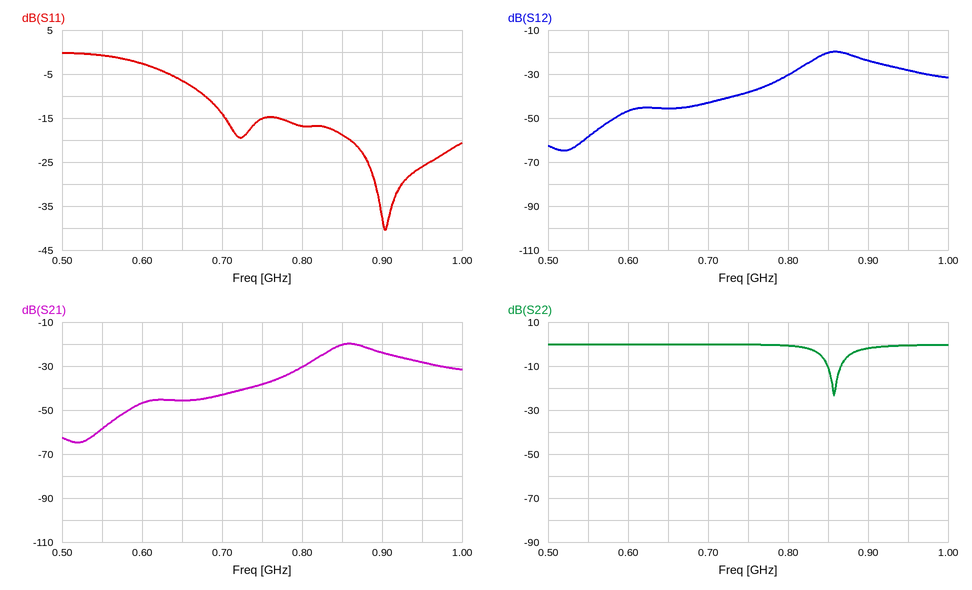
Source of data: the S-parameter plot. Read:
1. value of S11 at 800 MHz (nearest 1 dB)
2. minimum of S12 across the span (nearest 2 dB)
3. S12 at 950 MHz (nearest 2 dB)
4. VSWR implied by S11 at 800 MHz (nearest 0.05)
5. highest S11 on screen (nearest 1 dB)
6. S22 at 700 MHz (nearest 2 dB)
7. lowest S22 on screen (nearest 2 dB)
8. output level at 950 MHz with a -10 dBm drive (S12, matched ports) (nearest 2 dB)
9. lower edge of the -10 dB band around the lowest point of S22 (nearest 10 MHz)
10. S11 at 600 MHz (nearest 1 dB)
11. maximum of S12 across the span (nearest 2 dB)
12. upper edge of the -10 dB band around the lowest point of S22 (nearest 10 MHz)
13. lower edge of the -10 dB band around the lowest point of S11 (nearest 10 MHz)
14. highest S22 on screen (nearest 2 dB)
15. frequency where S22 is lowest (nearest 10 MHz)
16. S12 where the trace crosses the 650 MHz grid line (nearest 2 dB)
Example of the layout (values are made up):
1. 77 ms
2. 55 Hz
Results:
1. -17 dB
2. -64 dB
3. -28 dB
4. 1.35
5. 0 dB
6. 0 dB
7. -24 dB
8. -38 dBm
9. 850 MHz
10. -3 dB
11. -20 dB
12. 870 MHz
13. 680 MHz
14. 0 dB
15. 860 MHz
16. -46 dB
